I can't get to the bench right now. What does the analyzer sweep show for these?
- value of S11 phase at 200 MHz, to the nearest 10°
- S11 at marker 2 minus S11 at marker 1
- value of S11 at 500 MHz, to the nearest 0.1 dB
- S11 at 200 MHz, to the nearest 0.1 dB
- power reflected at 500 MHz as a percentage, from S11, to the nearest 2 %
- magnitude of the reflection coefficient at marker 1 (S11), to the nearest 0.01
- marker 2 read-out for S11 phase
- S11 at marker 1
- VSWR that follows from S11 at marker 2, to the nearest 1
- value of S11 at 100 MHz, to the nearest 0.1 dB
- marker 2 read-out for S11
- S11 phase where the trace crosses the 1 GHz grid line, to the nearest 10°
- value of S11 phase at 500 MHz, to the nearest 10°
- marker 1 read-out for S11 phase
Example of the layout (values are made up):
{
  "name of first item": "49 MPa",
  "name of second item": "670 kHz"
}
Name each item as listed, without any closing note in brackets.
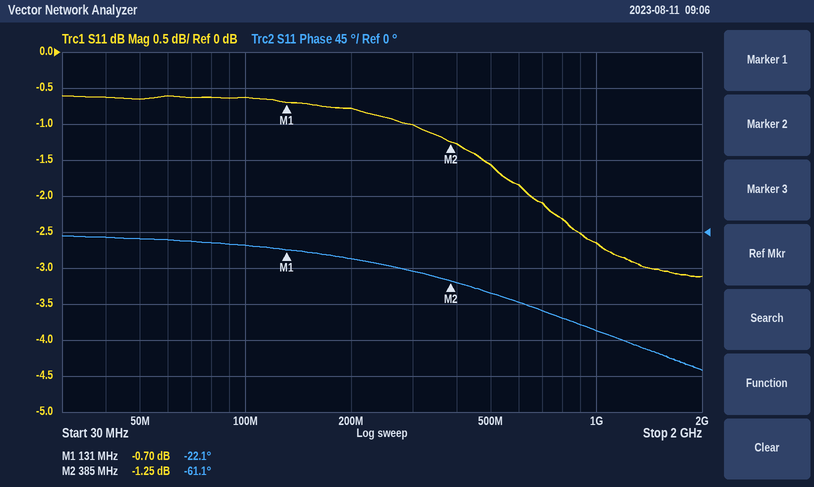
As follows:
{
  "value of S11 phase at 200 MHz, to the nearest 10°": "-30°",
  "S11 at marker 2 minus S11 at marker 1": "-0.55 dB",
  "value of S11 at 500 MHz, to the nearest 0.1 dB": "-1.6 dB",
  "S11 at 200 MHz, to the nearest 0.1 dB": "-0.8 dB",
  "power reflected at 500 MHz as a percentage, from S11, to the nearest 2 %": "70 %",
  "magnitude of the reflection coefficient at marker 1 (S11), to the nearest 0.01": "0.92",
  "marker 2 read-out for S11 phase": "-61.1°",
  "S11 at marker 1": "-0.70 dB",
  "VSWR that follows from S11 at marker 2, to the nearest 1": "14",
  "value of S11 at 100 MHz, to the nearest 0.1 dB": "-0.6 dB",
  "marker 2 read-out for S11": "-1.25 dB",
  "S11 phase where the trace crosses the 1 GHz grid line, to the nearest 10°": "-120°",
  "value of S11 phase at 500 MHz, to the nearest 10°": "-80°",
  "marker 1 read-out for S11 phase": "-22.1°"
}
